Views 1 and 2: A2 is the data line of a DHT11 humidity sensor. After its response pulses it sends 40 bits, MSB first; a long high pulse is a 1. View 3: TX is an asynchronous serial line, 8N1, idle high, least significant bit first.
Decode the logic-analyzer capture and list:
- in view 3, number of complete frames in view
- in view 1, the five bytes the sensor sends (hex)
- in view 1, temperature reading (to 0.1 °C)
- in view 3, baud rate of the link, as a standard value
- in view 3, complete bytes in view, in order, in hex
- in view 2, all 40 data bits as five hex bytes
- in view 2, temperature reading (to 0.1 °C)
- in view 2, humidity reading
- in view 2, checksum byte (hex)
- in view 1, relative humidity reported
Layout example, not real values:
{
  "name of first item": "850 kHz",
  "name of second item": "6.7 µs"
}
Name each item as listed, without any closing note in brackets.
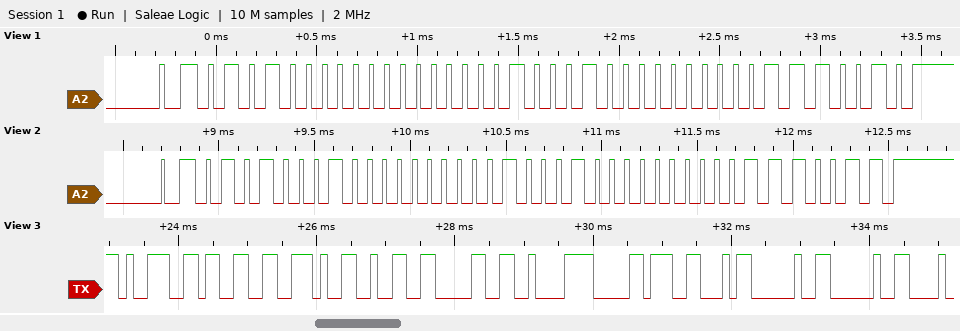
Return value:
{
  "in view 3, number of complete frames in view": "10",
  "in view 1, the five bytes the sensor sends": "50 00 22 00 72",
  "in view 1, temperature reading": "34.0 °C",
  "in view 3, baud rate of the link, as a standard value": "9600 baud",
  "in view 3, complete bytes in view, in order, in hex": "39 33 2E 32 30 C2 B0 46 20 20",
  "in view 2, all 40 data bits as five hex bytes": "51 00 22 00 73",
  "in view 2, temperature reading": "34.0 °C",
  "in view 2, humidity reading": "81 %",
  "in view 2, checksum byte": "0x73",
  "in view 1, relative humidity reported": "80 %"
}
